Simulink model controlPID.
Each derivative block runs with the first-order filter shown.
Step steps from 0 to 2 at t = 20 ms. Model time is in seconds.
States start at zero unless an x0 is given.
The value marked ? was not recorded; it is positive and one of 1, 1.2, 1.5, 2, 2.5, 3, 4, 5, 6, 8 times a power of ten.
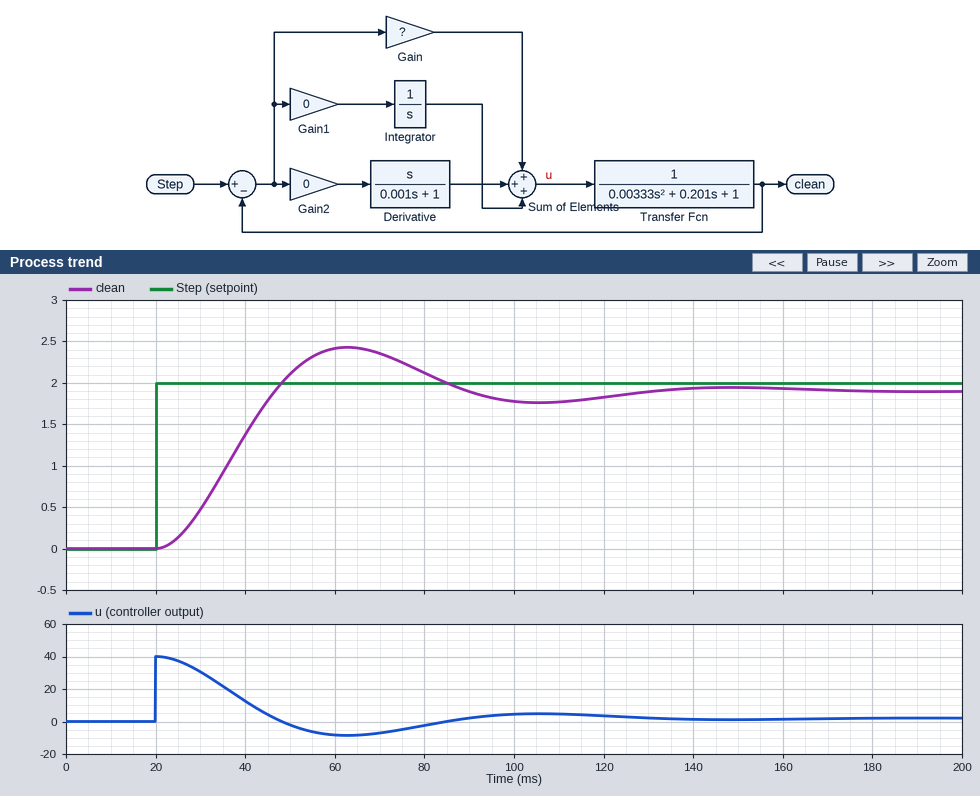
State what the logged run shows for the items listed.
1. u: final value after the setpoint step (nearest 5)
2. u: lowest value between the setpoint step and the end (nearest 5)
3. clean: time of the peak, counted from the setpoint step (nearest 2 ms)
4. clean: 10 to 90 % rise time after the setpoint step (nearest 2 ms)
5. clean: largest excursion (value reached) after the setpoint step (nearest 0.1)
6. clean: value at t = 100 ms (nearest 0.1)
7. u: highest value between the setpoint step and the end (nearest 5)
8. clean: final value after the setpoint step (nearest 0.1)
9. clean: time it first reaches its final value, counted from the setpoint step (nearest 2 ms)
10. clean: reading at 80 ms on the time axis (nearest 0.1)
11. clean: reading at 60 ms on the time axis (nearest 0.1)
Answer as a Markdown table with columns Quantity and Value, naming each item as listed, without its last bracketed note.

| Quantity | Value |
|---|---|
| u: final value after the setpoint step | 0 |
| u: lowest value between the setpoint step and the end | -10 |
| clean: time of the peak, counted from the setpoint step | 42 ms |
| clean: 10 to 90 % rise time after the setpoint step | 18 ms |
| clean: largest excursion (value reached) after the setpoint step | 2.4 |
| clean: value at t = 100 ms | 1.8 |
| u: highest value between the setpoint step and the end | 40 |
| clean: final value after the setpoint step | 1.9 |
| clean: time it first reaches its final value, counted from the setpoint step | 26 ms |
| clean: reading at 80 ms on the time axis | 2.1 |
| clean: reading at 60 ms on the time axis | 2.4 |
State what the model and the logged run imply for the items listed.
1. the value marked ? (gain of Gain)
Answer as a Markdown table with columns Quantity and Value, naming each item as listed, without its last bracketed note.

| Quantity | Value |
|---|---|
| the value marked ? | 20 |
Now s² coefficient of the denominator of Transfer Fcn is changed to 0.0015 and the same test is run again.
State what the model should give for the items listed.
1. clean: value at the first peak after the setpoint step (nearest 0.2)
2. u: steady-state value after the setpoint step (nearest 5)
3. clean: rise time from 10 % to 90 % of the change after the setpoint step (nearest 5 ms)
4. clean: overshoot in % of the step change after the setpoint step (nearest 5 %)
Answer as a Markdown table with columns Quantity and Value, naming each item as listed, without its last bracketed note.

| Quantity | Value |
|---|---|
| clean: value at the first peak after the setpoint step | 2.2 |
| u: steady-state value after the setpoint step | 0 |
| clean: rise time from 10 % to 90 % of the change after the setpoint step | 15 ms |
| clean: overshoot in % of the step change after the setpoint step | 10 % |
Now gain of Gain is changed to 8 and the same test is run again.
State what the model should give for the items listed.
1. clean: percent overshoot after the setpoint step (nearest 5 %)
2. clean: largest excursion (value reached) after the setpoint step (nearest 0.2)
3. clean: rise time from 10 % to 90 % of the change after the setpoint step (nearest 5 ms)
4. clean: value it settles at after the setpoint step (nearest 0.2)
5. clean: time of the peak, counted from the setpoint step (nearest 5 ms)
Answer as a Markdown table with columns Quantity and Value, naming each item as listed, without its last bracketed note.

| Quantity | Value |
|---|---|
| clean: percent overshoot after the setpoint step | 10 % |
| clean: largest excursion (value reached) after the setpoint step | 2.0 |
| clean: rise time from 10 % to 90 % of the change after the setpoint step | 35 ms |
| clean: value it settles at after the setpoint step | 1.8 |
| clean: time of the peak, counted from the setpoint step | 75 ms |
